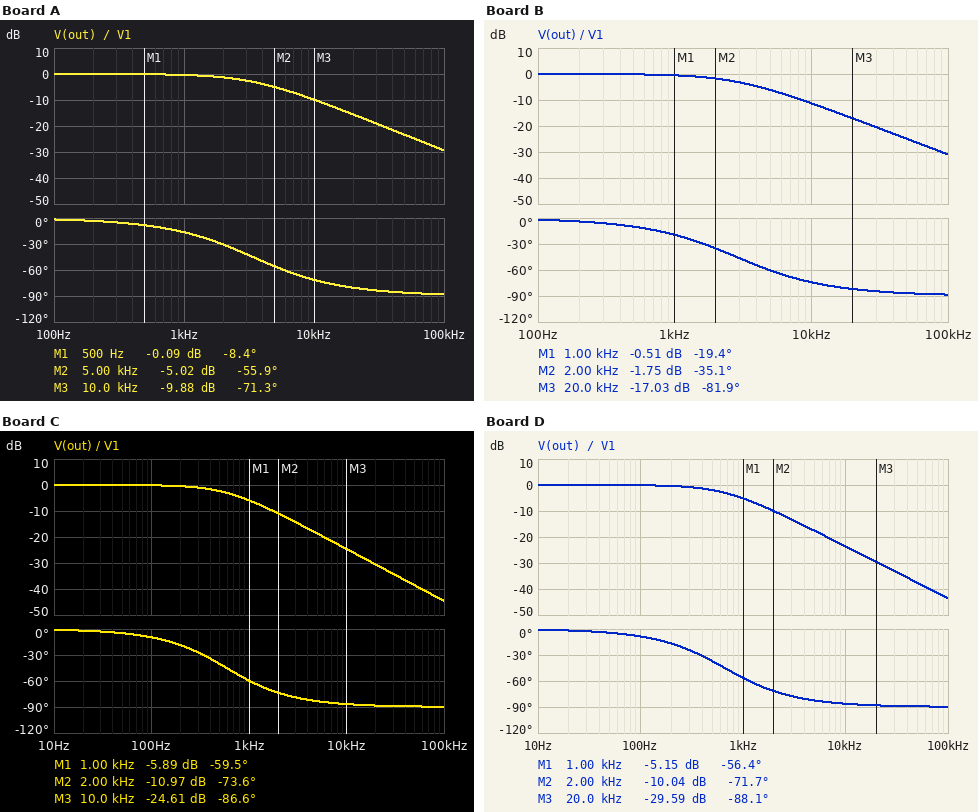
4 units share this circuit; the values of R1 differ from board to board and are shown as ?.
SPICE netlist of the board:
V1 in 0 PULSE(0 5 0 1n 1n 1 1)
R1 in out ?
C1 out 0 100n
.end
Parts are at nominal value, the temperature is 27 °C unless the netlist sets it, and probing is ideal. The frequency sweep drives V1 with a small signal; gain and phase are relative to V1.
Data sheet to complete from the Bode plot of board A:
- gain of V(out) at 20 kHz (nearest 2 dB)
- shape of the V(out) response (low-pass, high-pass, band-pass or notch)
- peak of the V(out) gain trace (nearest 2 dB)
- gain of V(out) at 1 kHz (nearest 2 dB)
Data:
-16 dB
low-pass
0 dB
0 dB
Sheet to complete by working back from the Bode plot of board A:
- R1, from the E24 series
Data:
470 Ω
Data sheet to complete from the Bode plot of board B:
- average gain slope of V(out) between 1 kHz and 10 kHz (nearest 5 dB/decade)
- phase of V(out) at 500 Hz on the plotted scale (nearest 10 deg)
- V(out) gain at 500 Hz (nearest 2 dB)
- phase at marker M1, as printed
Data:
-10 dB/decade
-10 deg
0 dB
-19.4 deg
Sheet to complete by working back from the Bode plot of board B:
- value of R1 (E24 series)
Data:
560 Ω
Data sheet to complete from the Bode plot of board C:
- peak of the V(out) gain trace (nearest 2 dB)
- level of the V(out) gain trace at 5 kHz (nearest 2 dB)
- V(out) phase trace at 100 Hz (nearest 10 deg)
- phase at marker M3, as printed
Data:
0 dB
-18 dB
-10 deg
-86.6 deg
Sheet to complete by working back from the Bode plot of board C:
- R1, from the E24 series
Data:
2.7 kΩ
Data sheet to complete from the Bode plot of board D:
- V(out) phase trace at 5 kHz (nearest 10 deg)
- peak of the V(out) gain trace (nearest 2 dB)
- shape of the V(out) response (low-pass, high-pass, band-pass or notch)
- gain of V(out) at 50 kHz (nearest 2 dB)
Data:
-80 deg
0 dB
low-pass
-38 dB
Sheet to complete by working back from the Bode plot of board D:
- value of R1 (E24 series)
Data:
2.4 kΩ
